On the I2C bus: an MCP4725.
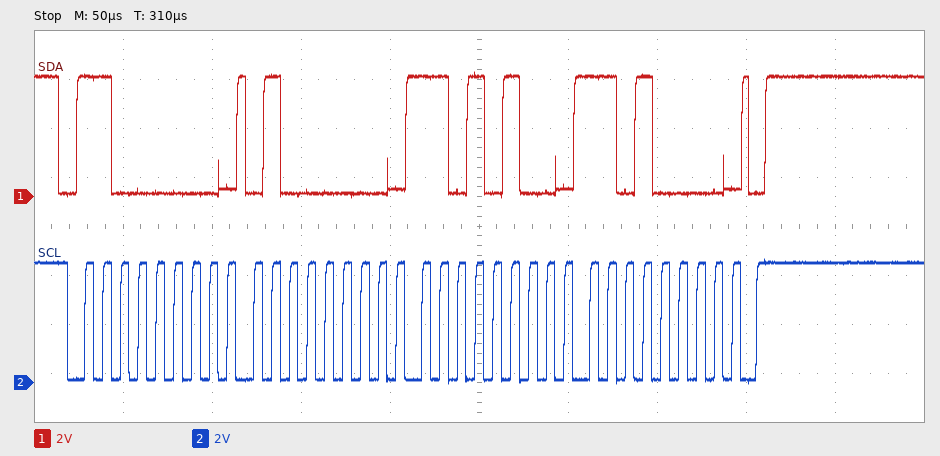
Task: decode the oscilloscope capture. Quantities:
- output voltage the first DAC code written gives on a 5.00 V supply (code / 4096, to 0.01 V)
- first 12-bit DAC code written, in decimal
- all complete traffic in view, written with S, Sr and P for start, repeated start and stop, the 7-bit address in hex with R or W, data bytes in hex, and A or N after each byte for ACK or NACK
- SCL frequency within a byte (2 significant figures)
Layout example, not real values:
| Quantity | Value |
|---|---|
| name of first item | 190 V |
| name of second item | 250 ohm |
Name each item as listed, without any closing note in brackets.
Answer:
| Quantity | Value |
|---|---|
| output voltage the first DAC code written gives on a 5.00 V supply | 4.16 V |
| first 12-bit DAC code written, in decimal | 3405 |
| all complete traffic in view, written with S, Sr and P for start, repeated start and stop, the 7-bit address in hex with R or W, data bytes in hex, and A or N after each byte for ACK or NACK | S 60W A 40 A D4 A D0 A P |
| SCL frequency within a byte | 100 kHz |
